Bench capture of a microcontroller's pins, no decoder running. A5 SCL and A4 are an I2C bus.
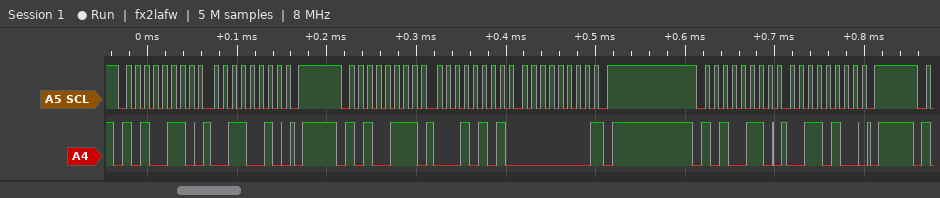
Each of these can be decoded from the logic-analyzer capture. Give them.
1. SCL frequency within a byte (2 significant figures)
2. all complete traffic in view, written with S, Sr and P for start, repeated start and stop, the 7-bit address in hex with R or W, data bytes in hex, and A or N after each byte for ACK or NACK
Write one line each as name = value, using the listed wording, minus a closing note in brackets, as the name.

SCL frequency within a byte = 100 kHz
all complete traffic in view, written with S, Sr and P for start, repeated start and stop, the 7-bit address in hex with R or W, data bytes in hex, and A or N after each byte for ACK or NACK = S 53W A 32 A P S 53R A 15 A 00 N P S 53W A 34 A P
